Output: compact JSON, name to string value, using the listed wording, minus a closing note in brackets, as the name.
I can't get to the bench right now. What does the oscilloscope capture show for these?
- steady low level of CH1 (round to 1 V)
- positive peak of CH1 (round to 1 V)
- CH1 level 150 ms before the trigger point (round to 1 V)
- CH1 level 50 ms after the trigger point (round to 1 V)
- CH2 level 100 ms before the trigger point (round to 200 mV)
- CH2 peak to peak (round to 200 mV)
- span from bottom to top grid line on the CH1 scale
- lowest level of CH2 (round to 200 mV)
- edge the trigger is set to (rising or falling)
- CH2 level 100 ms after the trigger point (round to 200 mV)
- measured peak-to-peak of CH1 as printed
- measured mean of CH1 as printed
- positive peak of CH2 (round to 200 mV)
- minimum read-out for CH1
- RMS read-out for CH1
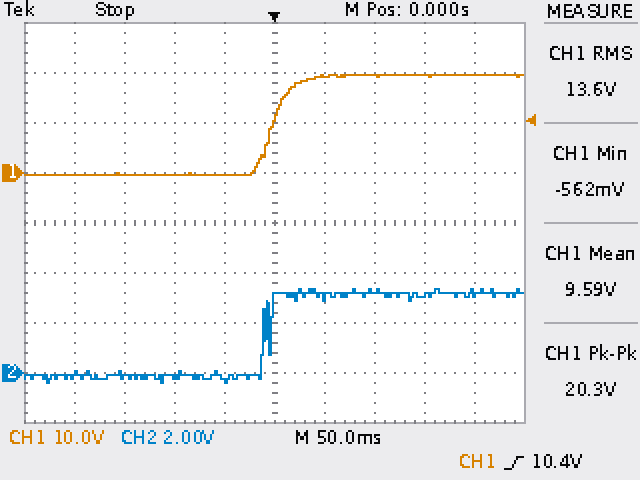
{"steady low level of CH1": "0 V", "positive peak of CH1": "20 V", "CH1 level 150 ms before the trigger point": "0 V", "CH1 level 50 ms after the trigger point": "19 V", "CH2 level 100 ms before the trigger point": "-200 mV", "CH2 peak to peak": "3.8 V", "span from bottom to top grid line on the CH1 scale": "80 V", "lowest level of CH2": "-400 mV", "edge the trigger is set to": "rising", "CH2 level 100 ms after the trigger point": "3.2 V", "measured peak-to-peak of CH1 as printed": "20.3 V", "measured mean of CH1 as printed": "9.59 V", "positive peak of CH2": "3.4 V", "minimum read-out for CH1": "-562 mV", "RMS read-out for CH1": "13.6 V"}
